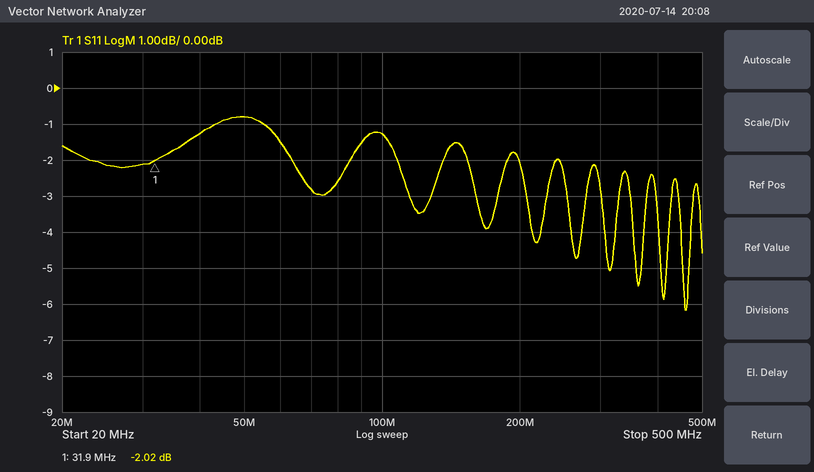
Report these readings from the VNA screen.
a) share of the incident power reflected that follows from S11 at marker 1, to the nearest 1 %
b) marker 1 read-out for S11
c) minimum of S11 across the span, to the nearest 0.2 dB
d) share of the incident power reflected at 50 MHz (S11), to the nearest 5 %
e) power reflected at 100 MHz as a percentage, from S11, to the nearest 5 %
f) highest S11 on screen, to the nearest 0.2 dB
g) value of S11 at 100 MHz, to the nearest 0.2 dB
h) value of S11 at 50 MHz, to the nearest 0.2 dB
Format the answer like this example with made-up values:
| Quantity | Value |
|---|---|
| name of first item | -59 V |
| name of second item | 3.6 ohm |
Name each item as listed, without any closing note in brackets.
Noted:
| Quantity | Value |
|---|---|
| share of the incident power reflected that follows from S11 at marker 1, to the nearest 1 % | 63 % |
| marker 1 read-out for S11 | -2.02 dB |
| minimum of S11 across the span, to the nearest 0.2 dB | -6.2 dB |
| share of the incident power reflected at 50 MHz (S11), to the nearest 5 % | 85 % |
| power reflected at 100 MHz as a percentage, from S11, to the nearest 5 % | 75 % |
| highest S11 on screen, to the nearest 0.2 dB | -0.8 dB |
| value of S11 at 100 MHz, to the nearest 0.2 dB | -1.2 dB |
| value of S11 at 50 MHz, to the nearest 0.2 dB | -0.8 dB |
